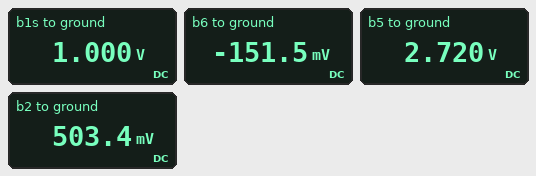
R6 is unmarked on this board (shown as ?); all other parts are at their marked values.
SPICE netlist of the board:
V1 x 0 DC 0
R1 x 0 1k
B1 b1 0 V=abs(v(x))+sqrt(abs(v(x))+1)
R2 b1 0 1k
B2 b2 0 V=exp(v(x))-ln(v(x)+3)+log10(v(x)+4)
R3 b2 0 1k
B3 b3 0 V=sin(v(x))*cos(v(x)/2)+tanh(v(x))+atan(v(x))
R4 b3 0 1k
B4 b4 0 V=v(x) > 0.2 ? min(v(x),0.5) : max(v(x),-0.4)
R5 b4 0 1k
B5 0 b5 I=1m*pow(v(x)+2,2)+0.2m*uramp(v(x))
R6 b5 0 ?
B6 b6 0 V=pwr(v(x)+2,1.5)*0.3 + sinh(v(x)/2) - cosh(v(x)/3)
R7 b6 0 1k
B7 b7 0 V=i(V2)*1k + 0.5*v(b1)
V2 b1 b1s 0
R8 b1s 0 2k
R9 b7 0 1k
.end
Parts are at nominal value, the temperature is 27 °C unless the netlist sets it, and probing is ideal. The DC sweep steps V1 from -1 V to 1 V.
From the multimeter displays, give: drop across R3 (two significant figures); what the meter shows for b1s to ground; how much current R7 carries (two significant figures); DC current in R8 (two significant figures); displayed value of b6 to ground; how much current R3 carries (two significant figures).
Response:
500 mV
1.000 V
150 µA
500 µA
-151.5 mV
500 µA
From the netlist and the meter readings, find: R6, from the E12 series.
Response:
680 Ω
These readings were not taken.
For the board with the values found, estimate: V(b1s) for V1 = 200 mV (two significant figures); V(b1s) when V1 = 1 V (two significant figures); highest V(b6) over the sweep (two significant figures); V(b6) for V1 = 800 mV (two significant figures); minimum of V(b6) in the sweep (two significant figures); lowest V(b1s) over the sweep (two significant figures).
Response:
1.3 V
2.4 V
1.0 V
780 mV
-1.3 V
1.0 V
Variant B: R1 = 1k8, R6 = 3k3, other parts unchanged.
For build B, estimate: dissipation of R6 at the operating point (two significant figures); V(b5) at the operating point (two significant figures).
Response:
53 mW
13 V
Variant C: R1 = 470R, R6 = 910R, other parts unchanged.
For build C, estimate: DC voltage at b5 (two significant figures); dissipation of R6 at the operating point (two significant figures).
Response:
3.6 V
15 mW
